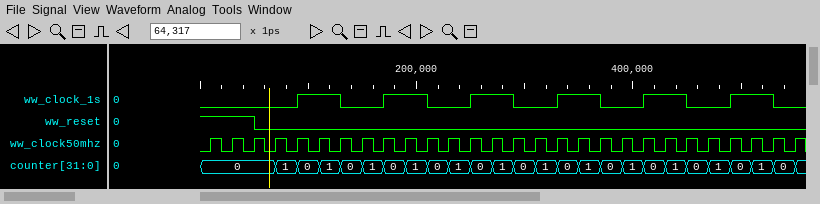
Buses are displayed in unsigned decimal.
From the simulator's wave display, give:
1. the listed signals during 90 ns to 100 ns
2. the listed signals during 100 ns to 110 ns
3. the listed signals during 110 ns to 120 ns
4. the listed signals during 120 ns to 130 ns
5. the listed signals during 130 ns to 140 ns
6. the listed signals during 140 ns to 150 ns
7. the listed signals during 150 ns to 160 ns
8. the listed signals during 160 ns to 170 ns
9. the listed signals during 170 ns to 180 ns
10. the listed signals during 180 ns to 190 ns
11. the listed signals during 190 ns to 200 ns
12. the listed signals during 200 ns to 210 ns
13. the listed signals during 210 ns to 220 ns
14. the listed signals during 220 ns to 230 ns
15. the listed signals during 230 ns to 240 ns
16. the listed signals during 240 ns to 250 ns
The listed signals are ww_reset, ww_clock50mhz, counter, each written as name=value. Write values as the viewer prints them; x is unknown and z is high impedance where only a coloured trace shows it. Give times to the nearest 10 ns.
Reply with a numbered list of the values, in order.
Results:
1. ww_reset=0, ww_clock50mhz=1, counter=0
2. ww_reset=0, ww_clock50mhz=0, counter=0
3. ww_reset=0, ww_clock50mhz=1, counter=1
4. ww_reset=0, ww_clock50mhz=0, counter=1
5. ww_reset=0, ww_clock50mhz=1, counter=0
6. ww_reset=0, ww_clock50mhz=0, counter=0
7. ww_reset=0, ww_clock50mhz=1, counter=1
8. ww_reset=0, ww_clock50mhz=0, counter=1
9. ww_reset=0, ww_clock50mhz=1, counter=0
10. ww_reset=0, ww_clock50mhz=0, counter=0
11. ww_reset=0, ww_clock50mhz=1, counter=1
12. ww_reset=0, ww_clock50mhz=0, counter=1
13. ww_reset=0, ww_clock50mhz=1, counter=0
14. ww_reset=0, ww_clock50mhz=0, counter=0
15. ww_reset=0, ww_clock50mhz=1, counter=1
16. ww_reset=0, ww_clock50mhz=0, counter=1
